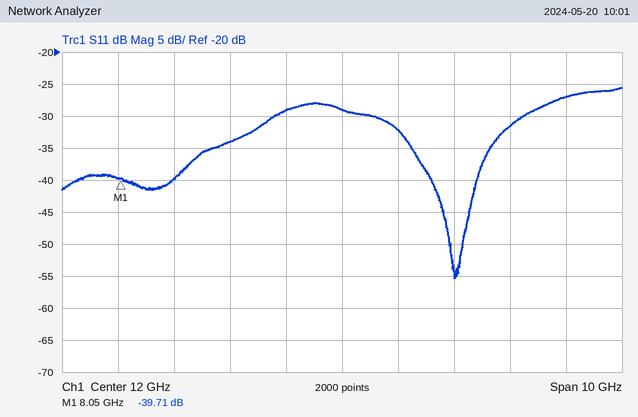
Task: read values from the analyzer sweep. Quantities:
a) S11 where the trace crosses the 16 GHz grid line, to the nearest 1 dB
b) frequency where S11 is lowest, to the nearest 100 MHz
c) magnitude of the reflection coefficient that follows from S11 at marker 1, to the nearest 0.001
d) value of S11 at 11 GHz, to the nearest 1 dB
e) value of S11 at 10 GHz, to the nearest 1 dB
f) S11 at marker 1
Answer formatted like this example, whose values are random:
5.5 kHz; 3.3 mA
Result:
-27 dB; 14.0 GHz; 0.010; -29 dB; -34 dB; -39.71 dB
